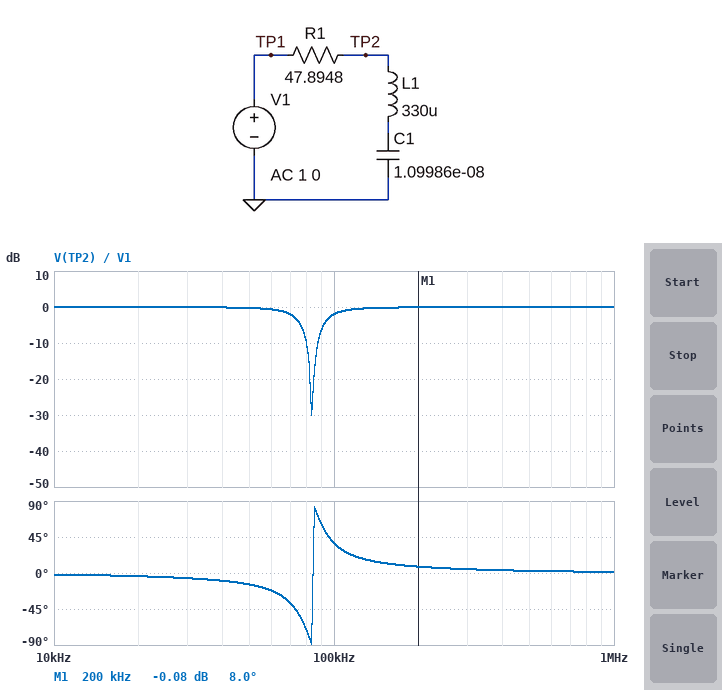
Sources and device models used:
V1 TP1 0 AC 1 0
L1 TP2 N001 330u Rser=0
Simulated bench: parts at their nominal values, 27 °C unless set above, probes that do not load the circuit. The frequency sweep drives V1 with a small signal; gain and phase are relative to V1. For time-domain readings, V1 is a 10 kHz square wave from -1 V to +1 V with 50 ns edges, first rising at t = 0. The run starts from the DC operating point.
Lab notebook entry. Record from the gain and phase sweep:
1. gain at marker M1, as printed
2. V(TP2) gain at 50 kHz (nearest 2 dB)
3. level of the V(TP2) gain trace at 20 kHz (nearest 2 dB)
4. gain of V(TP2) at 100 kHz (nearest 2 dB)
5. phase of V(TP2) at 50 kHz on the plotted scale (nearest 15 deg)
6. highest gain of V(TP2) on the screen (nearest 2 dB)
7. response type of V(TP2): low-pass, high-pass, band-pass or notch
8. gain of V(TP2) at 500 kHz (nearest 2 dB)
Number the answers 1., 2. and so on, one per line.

1. -0.08 dB
2. 0 dB
3. 0 dB
4. -2 dB
5. -15 deg
6. 0 dB
7. notch
8. 0 dB
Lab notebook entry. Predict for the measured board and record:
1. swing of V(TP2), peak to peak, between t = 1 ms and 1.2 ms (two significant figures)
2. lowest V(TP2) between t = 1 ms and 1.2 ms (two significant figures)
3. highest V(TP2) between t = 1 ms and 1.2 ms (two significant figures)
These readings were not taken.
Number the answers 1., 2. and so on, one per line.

1. 2.6 V
2. -1.3 V
3. 1.3 V
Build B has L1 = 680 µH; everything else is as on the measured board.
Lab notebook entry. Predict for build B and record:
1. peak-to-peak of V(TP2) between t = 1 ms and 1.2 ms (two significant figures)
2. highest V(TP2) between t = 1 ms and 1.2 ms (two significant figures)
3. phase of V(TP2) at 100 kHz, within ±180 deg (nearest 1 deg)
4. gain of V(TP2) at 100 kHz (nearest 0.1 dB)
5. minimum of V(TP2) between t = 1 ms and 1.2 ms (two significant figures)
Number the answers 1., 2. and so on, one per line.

1. 2.4 V
2. 1.2 V
3. 10 deg
4. -0.1 dB
5. -1.2 V
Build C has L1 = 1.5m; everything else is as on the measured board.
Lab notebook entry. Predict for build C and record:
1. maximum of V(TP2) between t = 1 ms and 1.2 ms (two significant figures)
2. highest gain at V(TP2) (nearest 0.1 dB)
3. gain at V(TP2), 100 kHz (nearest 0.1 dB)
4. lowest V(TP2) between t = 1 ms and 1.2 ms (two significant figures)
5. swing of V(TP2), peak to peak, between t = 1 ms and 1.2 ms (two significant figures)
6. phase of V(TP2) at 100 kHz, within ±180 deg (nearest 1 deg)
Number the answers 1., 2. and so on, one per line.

1. 1.1 V
2. 0 dB
3. 0 dB
4. -1.1 V
5. 2.3 V
6. 3 deg
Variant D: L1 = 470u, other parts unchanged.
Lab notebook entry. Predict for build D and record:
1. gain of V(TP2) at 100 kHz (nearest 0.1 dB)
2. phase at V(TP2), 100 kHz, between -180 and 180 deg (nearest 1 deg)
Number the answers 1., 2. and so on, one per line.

1. -0.4 dB
2. 18 deg
